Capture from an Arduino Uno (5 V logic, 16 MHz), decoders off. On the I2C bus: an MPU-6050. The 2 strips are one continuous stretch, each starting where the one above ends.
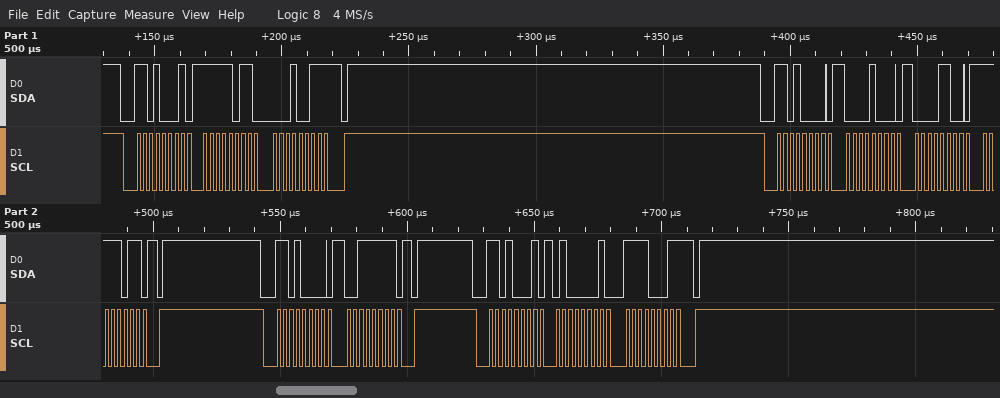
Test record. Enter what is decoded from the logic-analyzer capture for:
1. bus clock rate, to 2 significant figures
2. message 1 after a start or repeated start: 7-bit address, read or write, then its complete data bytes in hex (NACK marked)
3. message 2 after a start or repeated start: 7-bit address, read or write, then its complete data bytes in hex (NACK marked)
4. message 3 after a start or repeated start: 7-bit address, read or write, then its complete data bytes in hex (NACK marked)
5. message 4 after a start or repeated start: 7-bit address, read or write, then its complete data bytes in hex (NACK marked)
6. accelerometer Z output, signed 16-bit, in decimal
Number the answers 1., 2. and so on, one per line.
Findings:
1. 400 kHz
2. 0x68 read: FB 13 NACK
3. 0x68 write: 08 0C FB
4. 0x68 write: 3F
5. 0x68 read: 41 F1 NACK
6. 16881
